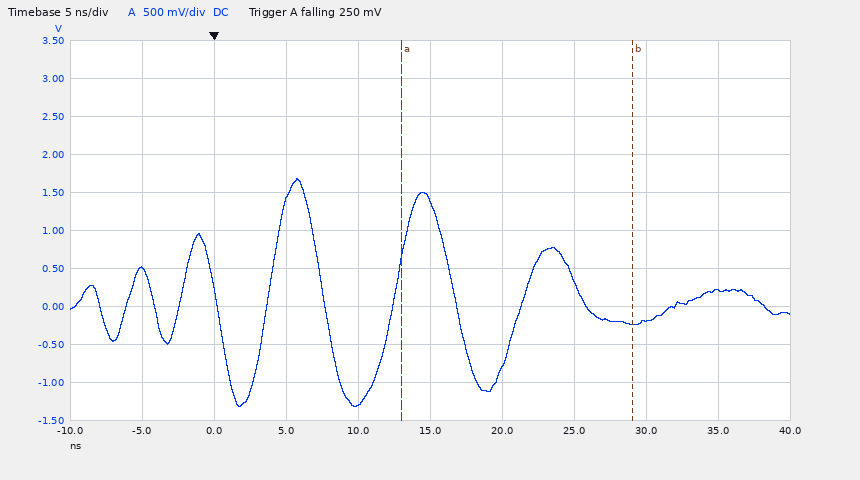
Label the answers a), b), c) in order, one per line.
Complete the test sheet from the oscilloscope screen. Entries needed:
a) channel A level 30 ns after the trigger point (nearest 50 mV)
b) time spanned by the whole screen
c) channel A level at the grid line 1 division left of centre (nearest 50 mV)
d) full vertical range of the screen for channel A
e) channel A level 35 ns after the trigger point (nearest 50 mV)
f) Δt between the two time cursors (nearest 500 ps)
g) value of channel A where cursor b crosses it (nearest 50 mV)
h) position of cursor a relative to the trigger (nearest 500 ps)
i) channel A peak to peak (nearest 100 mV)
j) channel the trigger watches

a) -200 mV
b) 50 ns
c) -1.30 V
d) 5 V
e) 200 mV
f) 16.0 ns
g) -250 mV
h) +13.0 ns
i) 3.00 V
j) channel A
